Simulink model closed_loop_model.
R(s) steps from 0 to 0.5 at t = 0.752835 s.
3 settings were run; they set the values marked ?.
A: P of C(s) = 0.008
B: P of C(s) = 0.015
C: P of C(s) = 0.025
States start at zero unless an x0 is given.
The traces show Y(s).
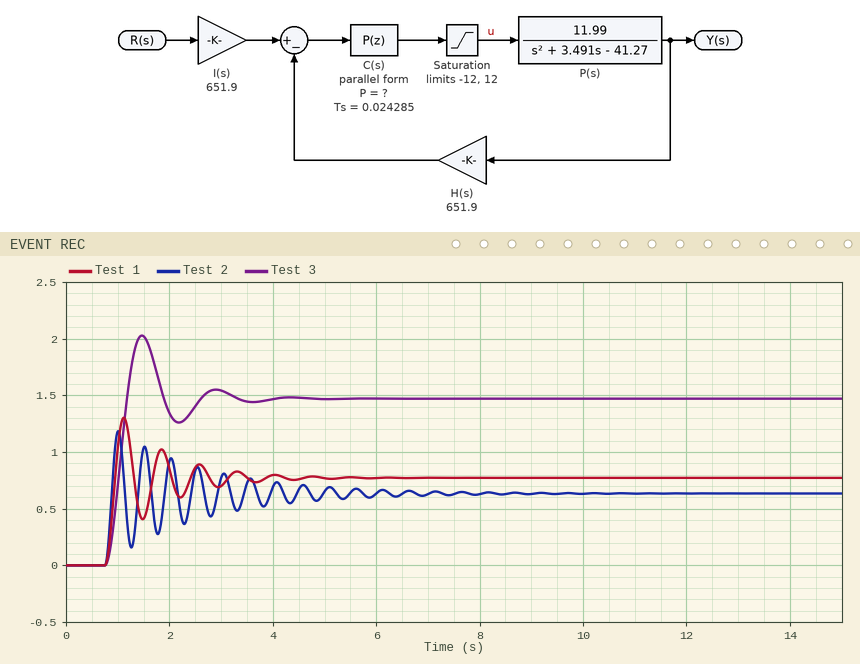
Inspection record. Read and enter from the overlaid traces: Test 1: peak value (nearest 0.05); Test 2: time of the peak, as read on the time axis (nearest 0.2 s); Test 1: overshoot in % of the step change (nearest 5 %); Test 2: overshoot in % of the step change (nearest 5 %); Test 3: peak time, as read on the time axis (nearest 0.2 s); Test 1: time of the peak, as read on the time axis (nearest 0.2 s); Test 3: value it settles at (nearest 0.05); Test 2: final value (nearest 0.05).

1.30
1.0 s
70 %
85 %
1.4 s
1.2 s
1.45
0.65
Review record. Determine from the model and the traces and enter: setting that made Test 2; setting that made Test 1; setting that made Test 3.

C
B
A
